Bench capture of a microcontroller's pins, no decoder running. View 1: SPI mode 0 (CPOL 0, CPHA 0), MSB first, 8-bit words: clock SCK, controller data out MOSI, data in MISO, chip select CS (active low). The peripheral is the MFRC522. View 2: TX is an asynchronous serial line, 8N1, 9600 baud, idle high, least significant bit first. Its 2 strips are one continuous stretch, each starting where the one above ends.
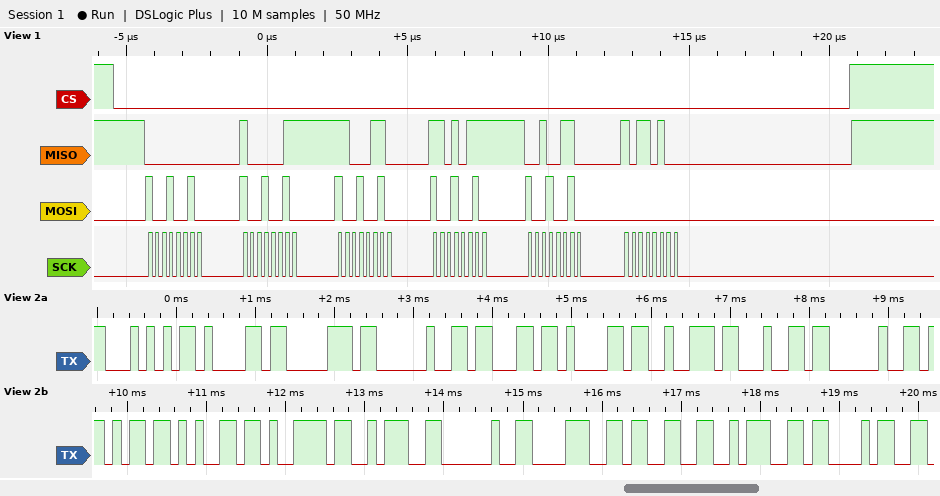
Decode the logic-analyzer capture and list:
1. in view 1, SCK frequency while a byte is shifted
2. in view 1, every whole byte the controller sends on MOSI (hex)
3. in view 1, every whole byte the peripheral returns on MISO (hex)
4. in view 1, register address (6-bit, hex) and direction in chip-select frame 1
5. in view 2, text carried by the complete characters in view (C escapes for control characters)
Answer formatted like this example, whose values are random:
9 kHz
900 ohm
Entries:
4 MHz
92 92 92 92 92 00
00 83 C6 D7 26 B4
0x09 read
"Tap card key: 83:C"
